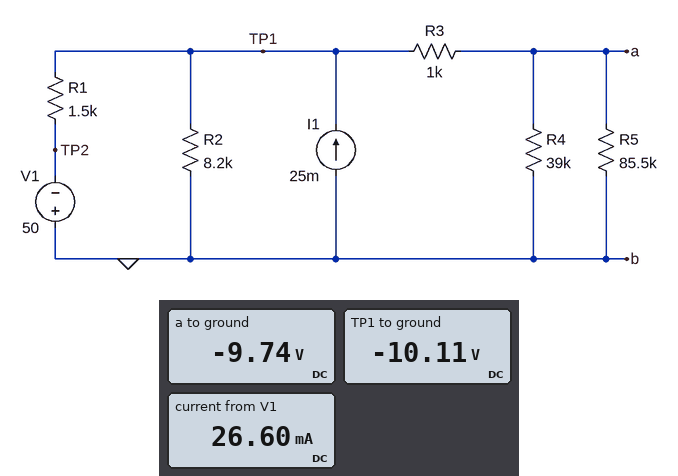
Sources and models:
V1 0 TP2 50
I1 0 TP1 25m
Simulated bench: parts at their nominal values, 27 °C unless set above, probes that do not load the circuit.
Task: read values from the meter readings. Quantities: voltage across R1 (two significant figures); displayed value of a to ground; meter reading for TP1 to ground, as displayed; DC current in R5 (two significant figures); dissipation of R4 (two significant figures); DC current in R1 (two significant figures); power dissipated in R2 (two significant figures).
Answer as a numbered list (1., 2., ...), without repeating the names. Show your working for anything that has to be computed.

1. -10.11 V - (-50 V) = 40 V
2. -9.74 V
3. -10.11 V
4. (0 V - (-9.74 V)) / 85.5 kΩ = 110 µA
5. (0 V - (-9.74 V))^2 / 39 kΩ = 2.4 mW
6. (-10.11 V - (-50 V)) / 1.5 kΩ = 27 mA
7. (0 V - (-10.11 V))^2 / 8.2 kΩ = 12 mW
